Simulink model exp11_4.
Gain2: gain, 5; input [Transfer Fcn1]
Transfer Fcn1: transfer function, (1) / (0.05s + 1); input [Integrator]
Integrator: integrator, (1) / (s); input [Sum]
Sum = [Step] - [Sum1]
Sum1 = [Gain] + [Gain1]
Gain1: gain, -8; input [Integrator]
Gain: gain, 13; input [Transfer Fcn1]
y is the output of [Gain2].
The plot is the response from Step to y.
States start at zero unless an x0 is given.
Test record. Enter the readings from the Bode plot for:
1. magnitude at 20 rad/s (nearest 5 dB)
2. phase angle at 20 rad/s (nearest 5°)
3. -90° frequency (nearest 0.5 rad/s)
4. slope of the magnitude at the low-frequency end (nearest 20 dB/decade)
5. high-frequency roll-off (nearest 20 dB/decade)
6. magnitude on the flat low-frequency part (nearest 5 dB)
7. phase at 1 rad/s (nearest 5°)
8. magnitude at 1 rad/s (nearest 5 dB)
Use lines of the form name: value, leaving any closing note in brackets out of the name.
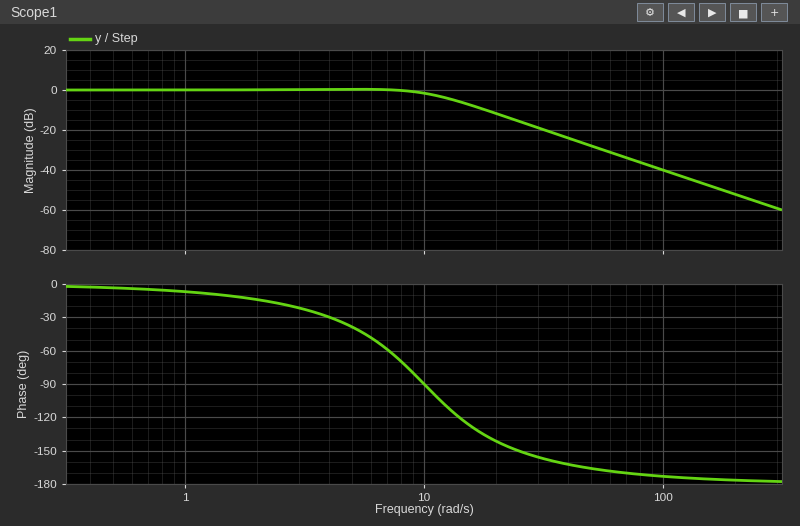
magnitude at 20 rad/s: -10 dB
phase angle at 20 rad/s: -140°
-90° frequency: 10.0 rad/s
slope of the magnitude at the low-frequency end: 0 dB/decade
high-frequency roll-off: -40 dB/decade
magnitude on the flat low-frequency part: 0 dB
phase at 1 rad/s: -5°
magnitude at 1 rad/s: 0 dB
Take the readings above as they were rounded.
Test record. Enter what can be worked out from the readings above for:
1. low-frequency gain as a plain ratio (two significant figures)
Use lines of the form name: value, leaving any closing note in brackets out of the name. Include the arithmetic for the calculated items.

low-frequency gain as a plain ratio: 10^(0 / 20) = 1.0
